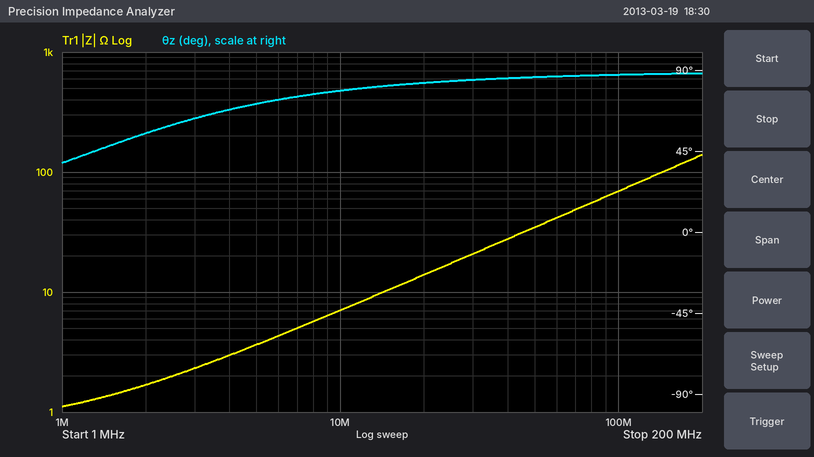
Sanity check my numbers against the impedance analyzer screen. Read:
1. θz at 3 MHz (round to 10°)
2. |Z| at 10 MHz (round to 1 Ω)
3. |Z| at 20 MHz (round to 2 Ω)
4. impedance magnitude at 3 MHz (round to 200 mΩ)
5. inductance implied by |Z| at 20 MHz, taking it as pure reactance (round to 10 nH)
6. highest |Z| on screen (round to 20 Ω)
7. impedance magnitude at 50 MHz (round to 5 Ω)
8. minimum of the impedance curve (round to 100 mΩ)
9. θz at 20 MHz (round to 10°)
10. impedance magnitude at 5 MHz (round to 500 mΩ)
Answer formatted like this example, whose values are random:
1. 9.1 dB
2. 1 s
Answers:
1. 60°
2. 7 Ω
3. 14 Ω
4. 2.4 Ω
5. 110 nH
6. 140 Ω
7. 35 Ω
8. 1.1 Ω
9. 80°
10. 3.5 Ω
